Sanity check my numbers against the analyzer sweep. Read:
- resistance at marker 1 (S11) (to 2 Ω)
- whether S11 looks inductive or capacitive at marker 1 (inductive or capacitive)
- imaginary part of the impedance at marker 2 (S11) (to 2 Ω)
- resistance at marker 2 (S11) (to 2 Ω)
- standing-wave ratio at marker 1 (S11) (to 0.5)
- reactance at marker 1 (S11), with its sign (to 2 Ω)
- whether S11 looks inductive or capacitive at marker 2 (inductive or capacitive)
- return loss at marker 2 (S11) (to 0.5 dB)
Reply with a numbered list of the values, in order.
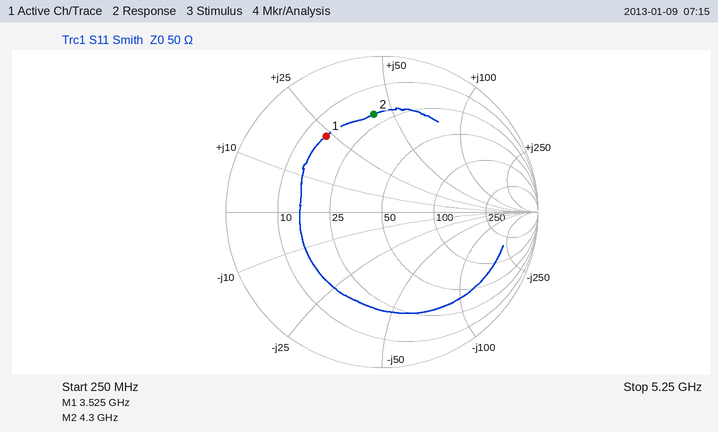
1. 16 Ω
2. inductive
3. +42 Ω
4. 20 Ω
5. 4.0
6. +24 Ω
7. inductive
8. 4.0 dB
